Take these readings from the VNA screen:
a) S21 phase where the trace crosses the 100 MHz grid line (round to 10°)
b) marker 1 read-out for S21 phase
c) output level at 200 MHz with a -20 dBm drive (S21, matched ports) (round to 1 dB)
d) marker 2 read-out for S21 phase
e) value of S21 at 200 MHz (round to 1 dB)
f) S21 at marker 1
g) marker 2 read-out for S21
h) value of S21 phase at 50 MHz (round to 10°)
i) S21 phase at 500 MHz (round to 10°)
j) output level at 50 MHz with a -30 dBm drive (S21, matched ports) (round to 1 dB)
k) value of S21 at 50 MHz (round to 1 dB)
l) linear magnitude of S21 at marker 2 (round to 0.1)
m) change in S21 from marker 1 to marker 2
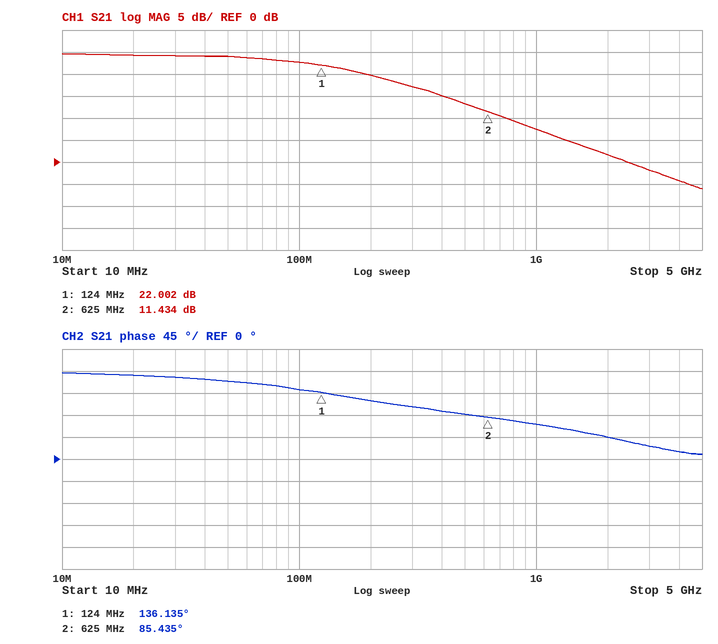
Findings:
140°
136.135°
0 dBm
85.435°
20 dB
22.002 dB
11.434 dB
160°
90°
-6 dBm
24 dB
3.7
-10.568 dB
